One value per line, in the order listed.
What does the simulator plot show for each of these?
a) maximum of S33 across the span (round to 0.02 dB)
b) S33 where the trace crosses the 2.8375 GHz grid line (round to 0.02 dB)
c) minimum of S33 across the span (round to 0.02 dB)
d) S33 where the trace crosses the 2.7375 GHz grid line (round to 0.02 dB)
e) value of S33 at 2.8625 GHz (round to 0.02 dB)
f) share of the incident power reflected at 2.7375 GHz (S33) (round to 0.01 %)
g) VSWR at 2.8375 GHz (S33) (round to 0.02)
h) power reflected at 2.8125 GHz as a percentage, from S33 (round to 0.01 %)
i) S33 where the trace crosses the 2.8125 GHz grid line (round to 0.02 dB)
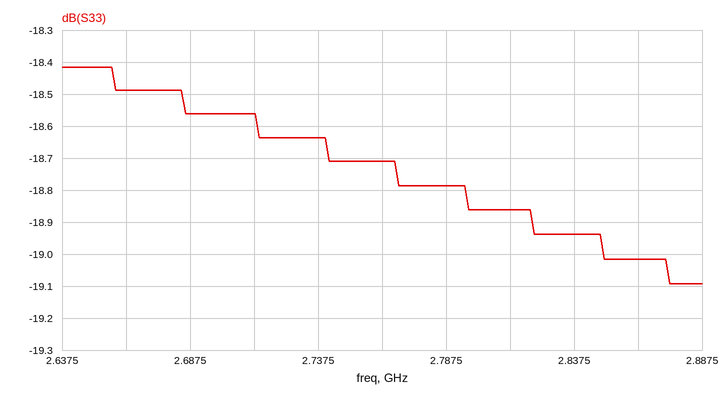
-18.42 dB
-18.94 dB
-19.10 dB
-18.64 dB
-19.02 dB
1.37 %
1.26
1.30 %
-18.86 dB
